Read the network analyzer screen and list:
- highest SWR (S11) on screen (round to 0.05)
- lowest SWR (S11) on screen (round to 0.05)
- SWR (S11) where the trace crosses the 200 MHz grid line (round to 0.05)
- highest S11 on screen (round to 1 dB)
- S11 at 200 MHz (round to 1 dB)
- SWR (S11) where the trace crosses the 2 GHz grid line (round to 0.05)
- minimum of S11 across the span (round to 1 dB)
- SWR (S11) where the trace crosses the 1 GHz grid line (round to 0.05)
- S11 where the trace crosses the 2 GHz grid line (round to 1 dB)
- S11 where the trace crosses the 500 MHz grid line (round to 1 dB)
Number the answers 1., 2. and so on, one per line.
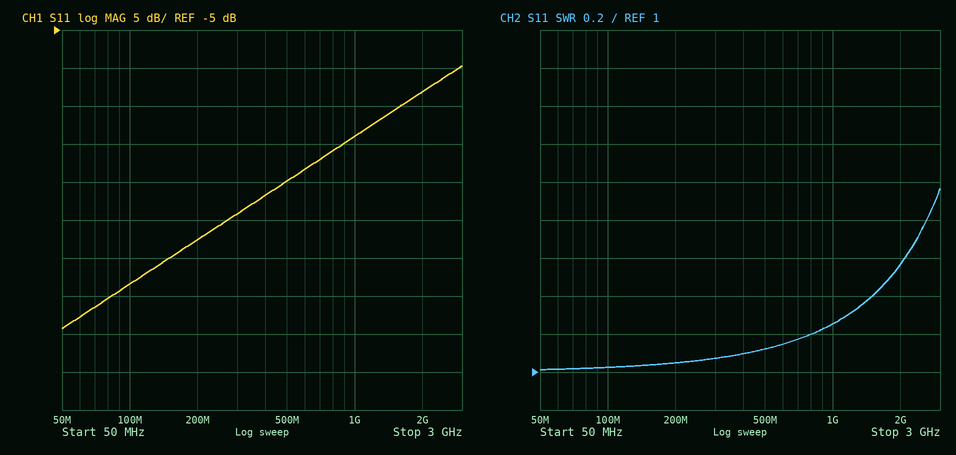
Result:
1. 1.95
2. 1.00
3. 1.05
4. -10 dB
5. -33 dB
6. 1.55
7. -44 dB
8. 1.25
9. -13 dB
10. -25 dB
